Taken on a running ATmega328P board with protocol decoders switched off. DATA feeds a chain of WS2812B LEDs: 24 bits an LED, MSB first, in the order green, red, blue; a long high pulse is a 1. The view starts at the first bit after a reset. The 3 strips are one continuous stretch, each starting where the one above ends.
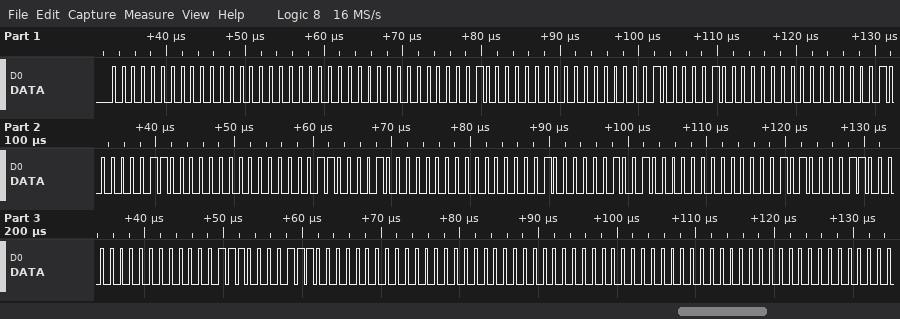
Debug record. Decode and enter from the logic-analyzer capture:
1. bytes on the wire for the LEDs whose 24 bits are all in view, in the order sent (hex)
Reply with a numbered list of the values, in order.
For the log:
1. 00 00 00 00 04 00 01 04 00 02 06 00 03 08 00 04 09 00 05 0C 00 07 0E 00 00 00 00 00 00 00
